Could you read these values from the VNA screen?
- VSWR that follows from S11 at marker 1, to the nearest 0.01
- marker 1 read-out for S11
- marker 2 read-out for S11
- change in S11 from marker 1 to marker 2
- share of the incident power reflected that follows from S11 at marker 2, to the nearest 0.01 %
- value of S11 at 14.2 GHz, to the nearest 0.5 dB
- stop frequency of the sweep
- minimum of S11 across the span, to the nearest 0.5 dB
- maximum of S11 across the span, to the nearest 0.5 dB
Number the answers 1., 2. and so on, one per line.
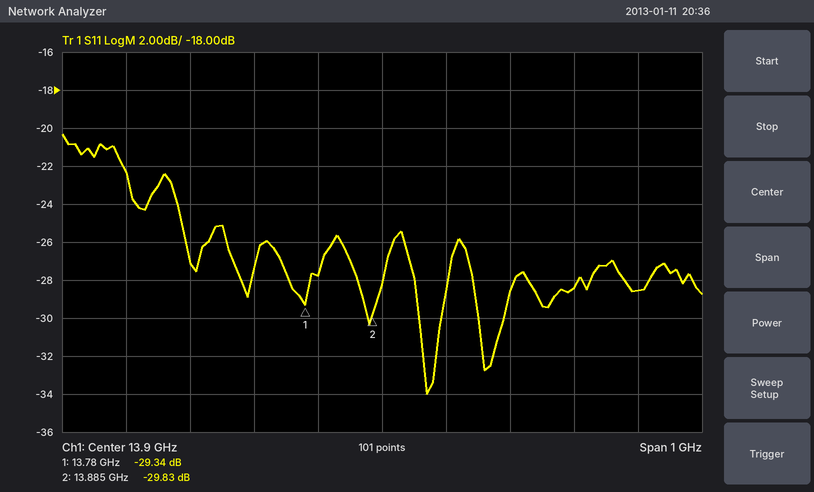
1. 1.07
2. -29.34 dB
3. -29.83 dB
4. -0.49 dB
5. 0.10 %
6. -28.5 dB
7. 14.4 GHz
8. -34.0 dB
9. -20.5 dB
